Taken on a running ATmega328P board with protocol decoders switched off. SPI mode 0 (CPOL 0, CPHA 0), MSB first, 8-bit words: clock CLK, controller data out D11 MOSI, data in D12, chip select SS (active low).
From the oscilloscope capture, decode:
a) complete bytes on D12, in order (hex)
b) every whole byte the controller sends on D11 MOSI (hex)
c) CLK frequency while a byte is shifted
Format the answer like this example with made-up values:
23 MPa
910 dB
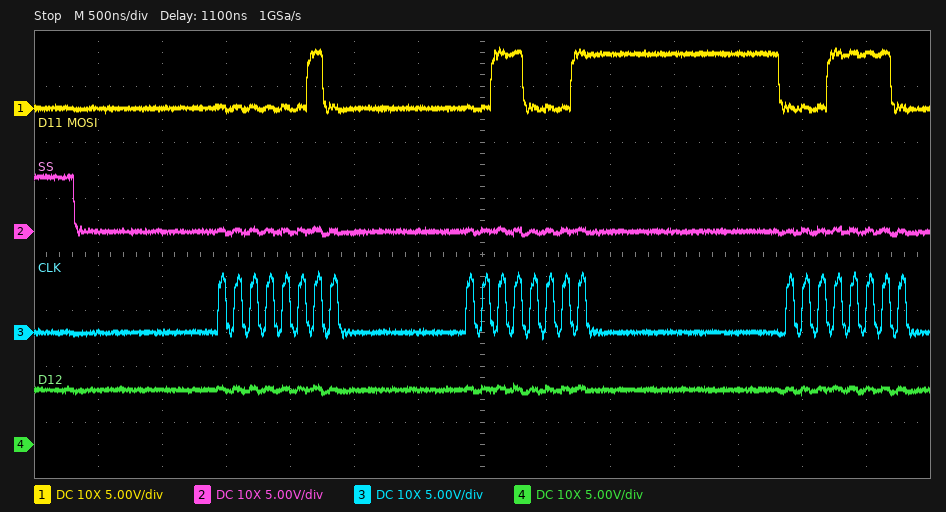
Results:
FF FF FF
02 31 1E
8 MHz
